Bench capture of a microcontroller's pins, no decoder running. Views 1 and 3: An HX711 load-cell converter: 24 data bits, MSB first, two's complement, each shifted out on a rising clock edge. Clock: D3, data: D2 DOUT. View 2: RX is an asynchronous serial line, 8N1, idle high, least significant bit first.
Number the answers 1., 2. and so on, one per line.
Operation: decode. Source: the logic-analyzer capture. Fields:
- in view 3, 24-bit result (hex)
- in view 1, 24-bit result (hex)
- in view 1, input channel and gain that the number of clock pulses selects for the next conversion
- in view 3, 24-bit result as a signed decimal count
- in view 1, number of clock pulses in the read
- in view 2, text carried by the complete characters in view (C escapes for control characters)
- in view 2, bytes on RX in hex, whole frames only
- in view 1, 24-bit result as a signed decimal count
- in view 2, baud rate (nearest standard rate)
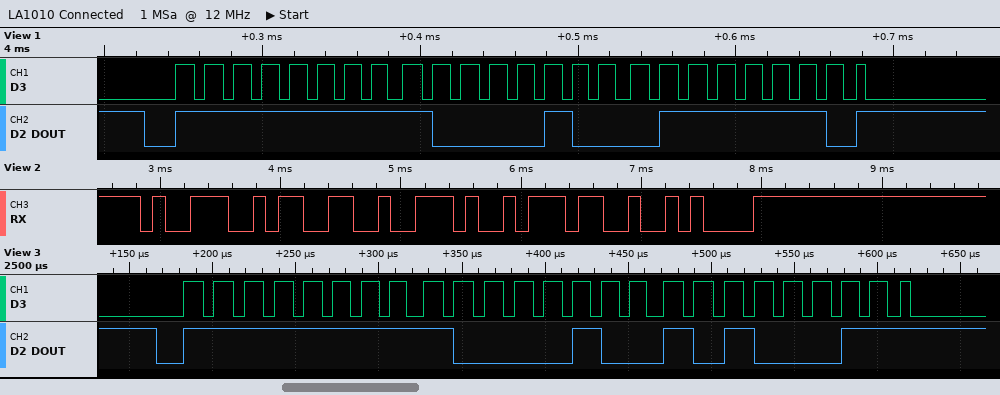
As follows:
1. 0xFF84A3
2. 0xFF847E
3. channel A, gain 128
4. -31581
5. 25
6. "93.7\n"
7. 39 33 2E 37 0A
8. -31618
9. 9600 baud
